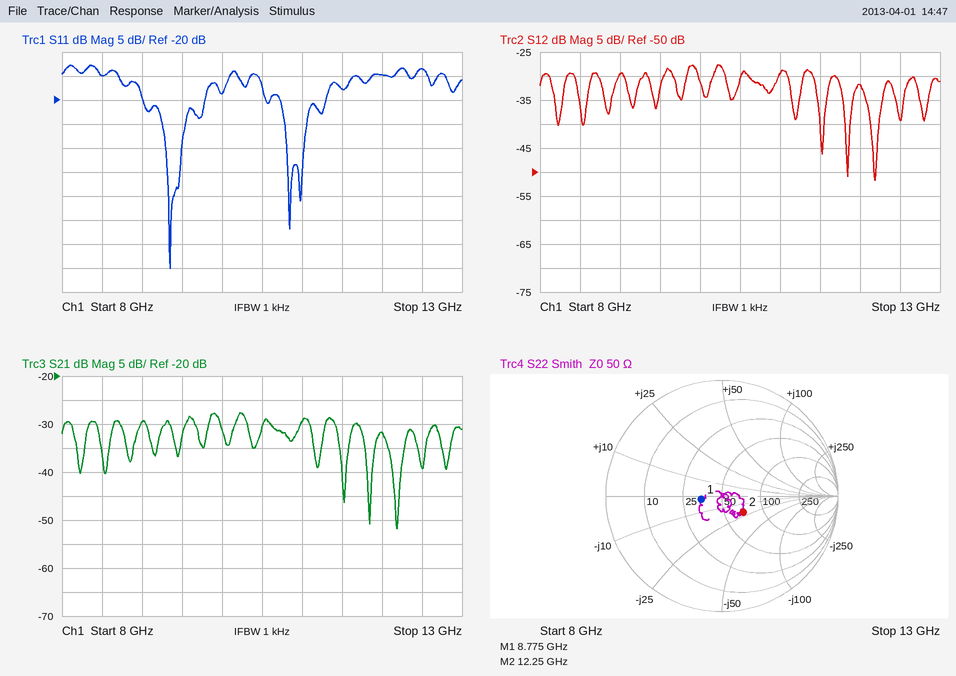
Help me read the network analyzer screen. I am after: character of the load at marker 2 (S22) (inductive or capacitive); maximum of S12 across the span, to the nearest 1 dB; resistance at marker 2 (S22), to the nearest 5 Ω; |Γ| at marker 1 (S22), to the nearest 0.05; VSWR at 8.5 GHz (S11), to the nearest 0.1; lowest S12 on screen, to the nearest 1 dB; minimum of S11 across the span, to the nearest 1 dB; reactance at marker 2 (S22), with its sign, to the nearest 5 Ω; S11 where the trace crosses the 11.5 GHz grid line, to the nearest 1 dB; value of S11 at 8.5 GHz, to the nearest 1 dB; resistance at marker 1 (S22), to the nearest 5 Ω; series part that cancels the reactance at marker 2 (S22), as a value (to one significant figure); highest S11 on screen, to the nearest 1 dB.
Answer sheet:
capacitive
-28 dB
70 Ω
0.20
1.4
-52 dB
-55 dB
-20 Ω
-18 dB
-15 dB
35 Ω
300 pH
-13 dB
